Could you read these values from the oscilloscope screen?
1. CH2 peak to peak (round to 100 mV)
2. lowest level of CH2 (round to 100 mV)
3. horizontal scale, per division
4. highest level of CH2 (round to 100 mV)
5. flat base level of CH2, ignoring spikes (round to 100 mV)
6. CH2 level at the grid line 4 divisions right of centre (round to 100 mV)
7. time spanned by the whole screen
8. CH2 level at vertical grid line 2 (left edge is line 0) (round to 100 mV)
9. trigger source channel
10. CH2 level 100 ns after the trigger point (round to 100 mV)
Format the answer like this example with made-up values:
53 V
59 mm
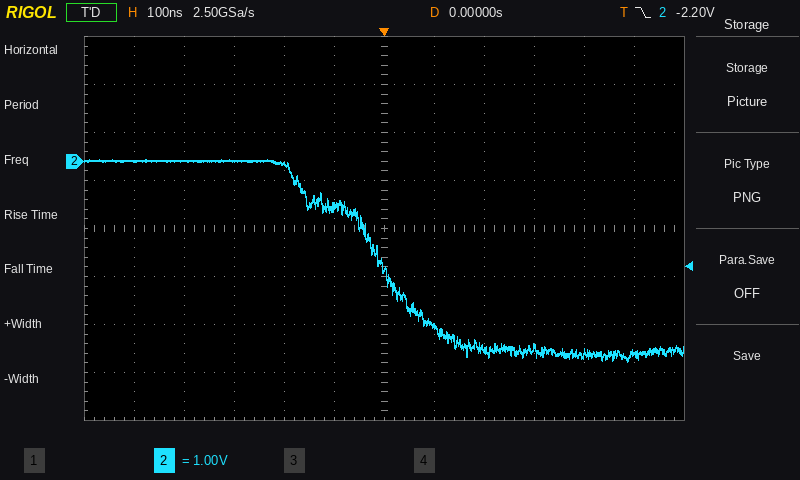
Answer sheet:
4.2 V
-4.2 V
100 ns
0.0 V
-4.0 V
-4.0 V
1.2 µs
0.0 V
CH2
-3.4 V
